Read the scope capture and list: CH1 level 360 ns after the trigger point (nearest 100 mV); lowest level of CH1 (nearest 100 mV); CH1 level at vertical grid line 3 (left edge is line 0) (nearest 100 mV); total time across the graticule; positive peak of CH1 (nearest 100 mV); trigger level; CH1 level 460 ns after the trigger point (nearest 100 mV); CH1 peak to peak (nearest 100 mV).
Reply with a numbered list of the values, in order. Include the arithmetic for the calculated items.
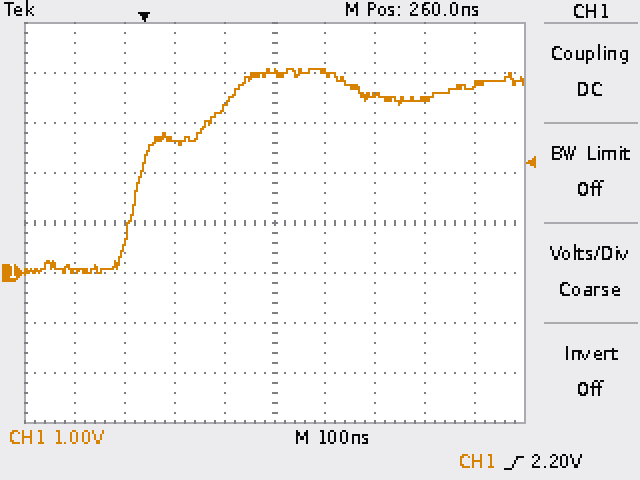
1. 4.0 V
2. 0.0 V
3. 2.7 V
4. 1 µs
5. 4.1 V
6. 2.20 V
7. 3.6 V
8. 4.1 V − (0.0 V) = 4.1 V
